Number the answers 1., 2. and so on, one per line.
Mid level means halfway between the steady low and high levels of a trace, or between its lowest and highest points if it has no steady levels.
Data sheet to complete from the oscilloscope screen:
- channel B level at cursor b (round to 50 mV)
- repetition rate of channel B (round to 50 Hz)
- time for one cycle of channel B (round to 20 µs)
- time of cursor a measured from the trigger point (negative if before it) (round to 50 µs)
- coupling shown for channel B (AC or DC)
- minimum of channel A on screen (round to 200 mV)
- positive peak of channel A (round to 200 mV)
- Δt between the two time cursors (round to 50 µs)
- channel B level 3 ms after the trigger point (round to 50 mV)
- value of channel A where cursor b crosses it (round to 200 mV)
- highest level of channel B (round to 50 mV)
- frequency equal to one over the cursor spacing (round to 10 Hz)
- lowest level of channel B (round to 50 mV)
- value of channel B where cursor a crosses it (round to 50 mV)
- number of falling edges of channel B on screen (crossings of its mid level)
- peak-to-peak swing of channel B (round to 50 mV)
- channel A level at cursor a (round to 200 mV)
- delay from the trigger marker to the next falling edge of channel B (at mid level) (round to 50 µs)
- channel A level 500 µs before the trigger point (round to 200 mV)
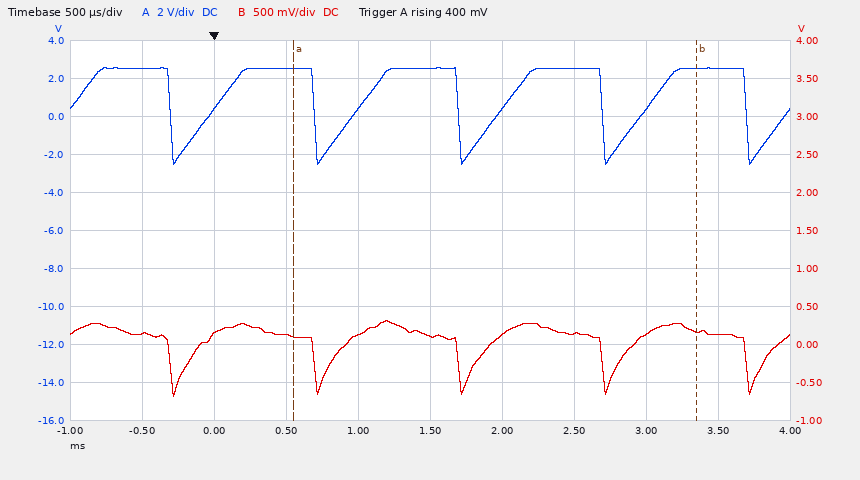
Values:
1. 150 mV
2. 1.00 kHz
3. 1.00 ms
4. +550 µs
5. DC
6. -2.6 V
7. 2.6 V
8. 2.80 ms
9. 150 mV
10. 2.6 V
11. 300 mV
12. 360 Hz
13. -700 mV
14. 100 mV
15. 5
16. 1.00 V
17. 2.6 V
18. 700 µs
19. 2.6 V
